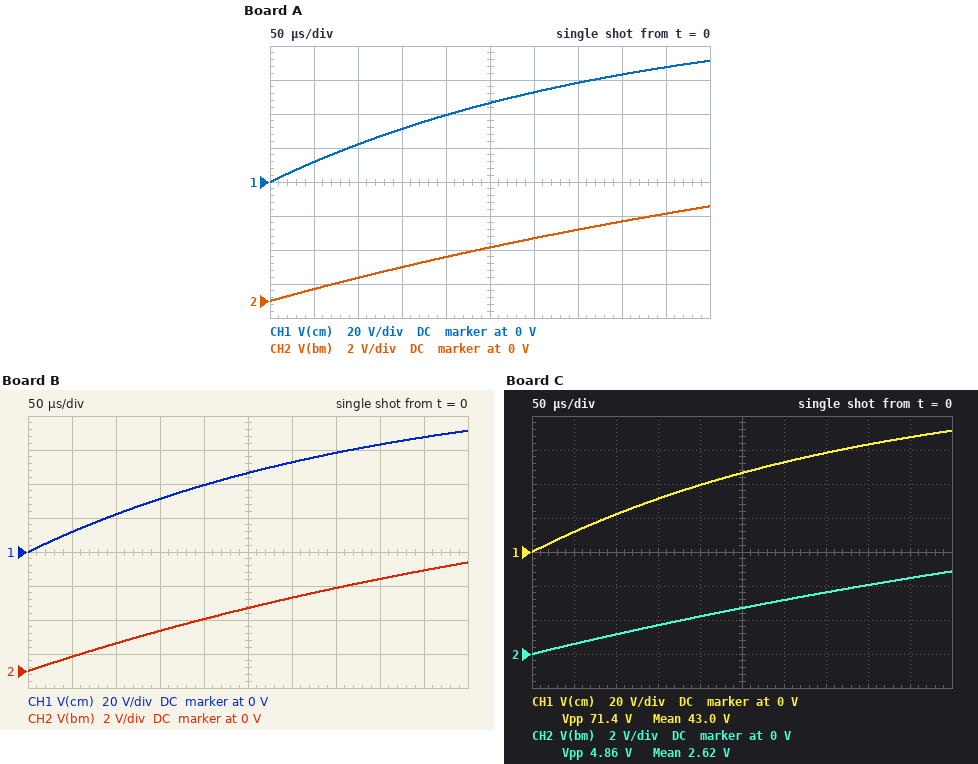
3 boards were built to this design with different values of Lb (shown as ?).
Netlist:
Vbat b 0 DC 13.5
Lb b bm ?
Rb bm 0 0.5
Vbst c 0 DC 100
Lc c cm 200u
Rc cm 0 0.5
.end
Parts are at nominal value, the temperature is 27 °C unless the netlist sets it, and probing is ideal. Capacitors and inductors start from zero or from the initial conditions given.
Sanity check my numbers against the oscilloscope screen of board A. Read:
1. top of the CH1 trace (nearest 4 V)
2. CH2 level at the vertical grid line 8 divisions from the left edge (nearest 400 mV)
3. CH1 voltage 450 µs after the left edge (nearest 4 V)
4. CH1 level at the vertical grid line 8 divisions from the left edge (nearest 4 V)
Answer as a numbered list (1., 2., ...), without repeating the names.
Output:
1. 72 V
2. 4.8 V
3. 68 V
4. 64 V
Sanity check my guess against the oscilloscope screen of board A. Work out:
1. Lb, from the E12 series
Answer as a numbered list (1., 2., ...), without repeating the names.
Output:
1. 470 µH
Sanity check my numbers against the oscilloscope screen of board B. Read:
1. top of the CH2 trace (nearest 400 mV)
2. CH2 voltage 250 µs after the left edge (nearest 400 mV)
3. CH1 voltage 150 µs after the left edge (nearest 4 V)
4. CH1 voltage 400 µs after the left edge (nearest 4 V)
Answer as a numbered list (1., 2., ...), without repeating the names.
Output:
1. 6.4 V
2. 3.6 V
3. 32 V
4. 64 V
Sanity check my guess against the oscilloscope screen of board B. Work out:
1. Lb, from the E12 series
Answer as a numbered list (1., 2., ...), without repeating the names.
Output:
1. 390 µH
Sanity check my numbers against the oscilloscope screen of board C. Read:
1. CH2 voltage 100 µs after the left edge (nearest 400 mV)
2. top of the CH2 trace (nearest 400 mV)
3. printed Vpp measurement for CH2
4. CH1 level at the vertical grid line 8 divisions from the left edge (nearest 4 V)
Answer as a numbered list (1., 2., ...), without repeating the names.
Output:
1. 1.2 V
2. 4.8 V
3. 4.86 V
4. 64 V
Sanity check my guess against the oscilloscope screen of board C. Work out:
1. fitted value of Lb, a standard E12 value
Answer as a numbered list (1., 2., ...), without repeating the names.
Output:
1. 560 µH
